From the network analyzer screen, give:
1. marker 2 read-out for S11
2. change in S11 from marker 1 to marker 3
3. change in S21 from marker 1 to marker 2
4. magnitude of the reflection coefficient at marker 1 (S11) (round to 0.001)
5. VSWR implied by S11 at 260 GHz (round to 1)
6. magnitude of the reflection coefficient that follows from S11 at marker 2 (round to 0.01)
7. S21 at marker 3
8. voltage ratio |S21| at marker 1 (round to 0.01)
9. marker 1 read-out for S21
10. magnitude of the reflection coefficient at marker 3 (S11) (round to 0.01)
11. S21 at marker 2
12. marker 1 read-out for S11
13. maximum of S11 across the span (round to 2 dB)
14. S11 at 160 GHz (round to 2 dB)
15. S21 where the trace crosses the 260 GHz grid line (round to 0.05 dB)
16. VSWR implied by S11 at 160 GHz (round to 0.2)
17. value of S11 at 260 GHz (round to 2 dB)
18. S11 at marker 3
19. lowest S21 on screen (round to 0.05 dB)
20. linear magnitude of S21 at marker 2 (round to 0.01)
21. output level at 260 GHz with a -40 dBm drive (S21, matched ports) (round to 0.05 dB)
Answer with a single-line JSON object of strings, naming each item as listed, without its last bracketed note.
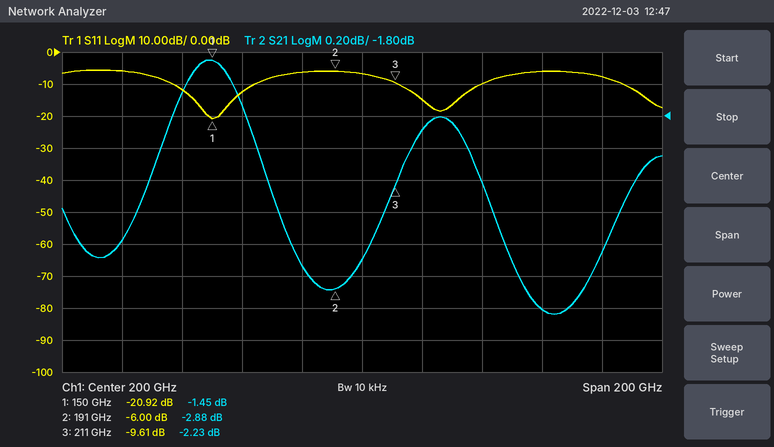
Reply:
{"marker 2 read-out for S11": "-6.00 dB", "change in S11 from marker 1 to marker 3": "11.31 dB", "change in S21 from marker 1 to marker 2": "-1.43 dB", "magnitude of the reflection coefficient at marker 1 (S11)": "0.090", "VSWR implied by S11 at 260 GHz": "3", "magnitude of the reflection coefficient that follows from S11 at marker 2": "0.50", "S21 at marker 3": "-2.23 dB", "voltage ratio |S21| at marker 1": "0.85", "marker 1 read-out for S21": "-1.45 dB", "magnitude of the reflection coefficient at marker 3 (S11)": "0.33", "S21 at marker 2": "-2.88 dB", "marker 1 read-out for S11": "-20.92 dB", "maximum of S11 across the span": "-6 dB", "S11 at 160 GHz": "-12 dB", "S21 where the trace crosses the 260 GHz grid line": "-3.00 dB", "VSWR implied by S11 at 160 GHz": "1.6", "value of S11 at 260 GHz": "-6 dB", "S11 at marker 3": "-9.61 dB", "lowest S21 on screen": "-3.05 dB", "linear magnitude of S21 at marker 2": "0.72", "output level at 260 GHz with a -40 dBm drive (S21, matched ports)": "-43.00 dBm"}
